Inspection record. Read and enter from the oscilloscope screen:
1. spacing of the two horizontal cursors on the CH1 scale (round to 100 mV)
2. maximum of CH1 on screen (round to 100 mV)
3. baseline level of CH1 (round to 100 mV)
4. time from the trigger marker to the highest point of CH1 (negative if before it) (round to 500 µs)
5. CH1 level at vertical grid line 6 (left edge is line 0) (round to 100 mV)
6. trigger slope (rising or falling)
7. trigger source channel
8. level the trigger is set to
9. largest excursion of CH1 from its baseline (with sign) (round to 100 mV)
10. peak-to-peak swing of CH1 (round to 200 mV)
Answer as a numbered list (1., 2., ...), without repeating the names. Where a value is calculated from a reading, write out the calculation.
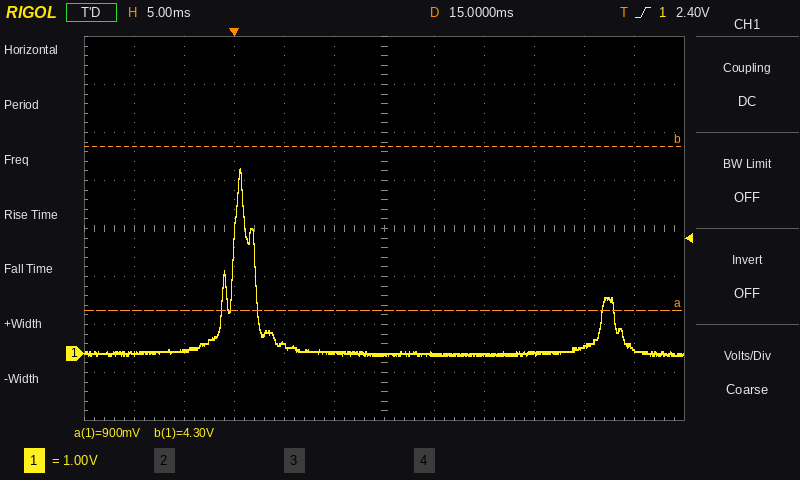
1. 3.4 V
2. 3.8 V
3. 0.0 V
4. +500 µs
5. 0.0 V
6. rising
7. CH1
8. 2.40 V
9. 3.8 V − (0.0 V) = +3.8 V
10. 3.8 V
